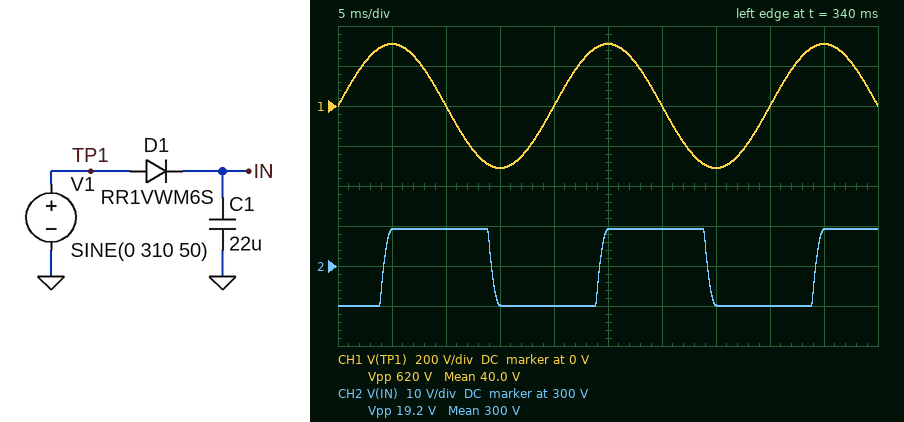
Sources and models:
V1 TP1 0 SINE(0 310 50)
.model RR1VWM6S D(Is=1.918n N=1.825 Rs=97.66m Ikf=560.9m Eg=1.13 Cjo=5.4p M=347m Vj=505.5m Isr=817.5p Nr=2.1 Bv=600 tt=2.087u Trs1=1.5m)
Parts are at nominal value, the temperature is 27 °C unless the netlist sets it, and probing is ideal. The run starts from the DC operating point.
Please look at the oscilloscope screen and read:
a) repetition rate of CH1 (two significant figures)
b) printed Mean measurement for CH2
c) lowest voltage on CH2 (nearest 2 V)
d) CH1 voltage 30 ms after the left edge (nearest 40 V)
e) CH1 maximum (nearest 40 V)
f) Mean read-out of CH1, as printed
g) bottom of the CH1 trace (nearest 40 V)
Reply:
50 Hz
300 V
290 V
0 V
320 V
40.0 V
-320 V
